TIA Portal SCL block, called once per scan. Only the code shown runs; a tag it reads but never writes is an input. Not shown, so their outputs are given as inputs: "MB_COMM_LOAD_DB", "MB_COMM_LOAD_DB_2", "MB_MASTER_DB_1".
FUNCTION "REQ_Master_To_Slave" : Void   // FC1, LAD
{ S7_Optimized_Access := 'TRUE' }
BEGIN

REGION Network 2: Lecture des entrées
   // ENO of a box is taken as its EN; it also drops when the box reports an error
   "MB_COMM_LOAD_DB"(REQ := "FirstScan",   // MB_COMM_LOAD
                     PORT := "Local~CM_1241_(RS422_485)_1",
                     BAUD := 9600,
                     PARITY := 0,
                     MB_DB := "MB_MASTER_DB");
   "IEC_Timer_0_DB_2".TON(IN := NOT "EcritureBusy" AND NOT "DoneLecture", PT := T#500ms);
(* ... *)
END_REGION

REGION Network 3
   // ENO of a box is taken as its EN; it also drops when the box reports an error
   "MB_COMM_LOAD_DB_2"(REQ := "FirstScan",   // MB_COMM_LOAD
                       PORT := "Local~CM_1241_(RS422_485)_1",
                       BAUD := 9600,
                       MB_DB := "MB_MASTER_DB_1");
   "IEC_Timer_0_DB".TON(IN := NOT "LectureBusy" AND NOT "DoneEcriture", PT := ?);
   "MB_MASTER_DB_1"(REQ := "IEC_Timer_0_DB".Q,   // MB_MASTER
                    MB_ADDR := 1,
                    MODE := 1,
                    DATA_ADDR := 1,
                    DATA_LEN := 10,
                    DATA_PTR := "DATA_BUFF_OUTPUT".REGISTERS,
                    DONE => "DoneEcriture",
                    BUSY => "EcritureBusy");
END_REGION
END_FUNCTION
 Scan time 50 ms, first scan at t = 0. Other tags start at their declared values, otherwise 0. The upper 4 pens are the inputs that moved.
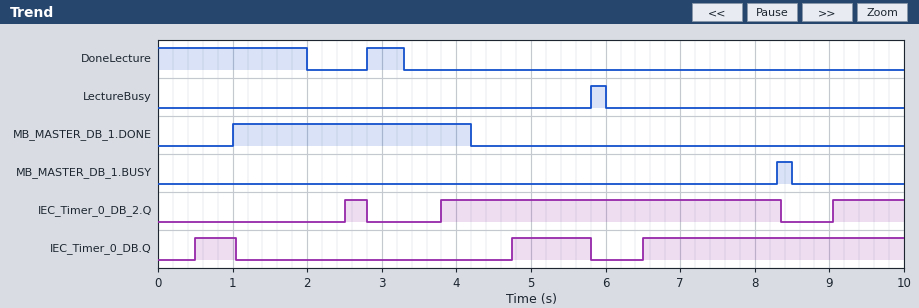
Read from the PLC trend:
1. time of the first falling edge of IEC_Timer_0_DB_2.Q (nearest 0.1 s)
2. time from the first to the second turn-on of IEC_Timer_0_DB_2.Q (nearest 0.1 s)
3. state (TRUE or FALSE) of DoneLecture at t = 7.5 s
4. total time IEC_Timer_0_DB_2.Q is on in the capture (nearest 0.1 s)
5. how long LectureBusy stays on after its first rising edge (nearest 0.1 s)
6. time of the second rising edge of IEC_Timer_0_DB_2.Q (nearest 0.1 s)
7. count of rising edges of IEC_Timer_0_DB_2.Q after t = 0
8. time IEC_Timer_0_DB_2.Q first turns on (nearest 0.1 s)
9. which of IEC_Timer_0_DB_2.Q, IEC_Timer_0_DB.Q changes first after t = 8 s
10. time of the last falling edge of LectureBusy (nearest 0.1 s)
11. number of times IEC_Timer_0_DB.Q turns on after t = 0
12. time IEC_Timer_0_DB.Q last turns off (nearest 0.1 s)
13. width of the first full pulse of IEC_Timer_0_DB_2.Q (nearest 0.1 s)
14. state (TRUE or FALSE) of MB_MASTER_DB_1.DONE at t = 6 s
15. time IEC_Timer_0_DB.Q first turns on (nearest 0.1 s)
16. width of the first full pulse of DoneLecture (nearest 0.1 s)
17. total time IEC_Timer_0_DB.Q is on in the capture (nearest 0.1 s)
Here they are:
2.8 s
1.3 s
FALSE
5.8 s
0.2 s
3.8 s
3
2.5 s
IEC_Timer_0_DB_2.Q
6.0 s
3
5.8 s
0.3 s
FALSE
0.5 s
0.5 s
5.1 s
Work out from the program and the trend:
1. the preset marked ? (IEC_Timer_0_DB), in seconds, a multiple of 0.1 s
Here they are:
0.5 s
